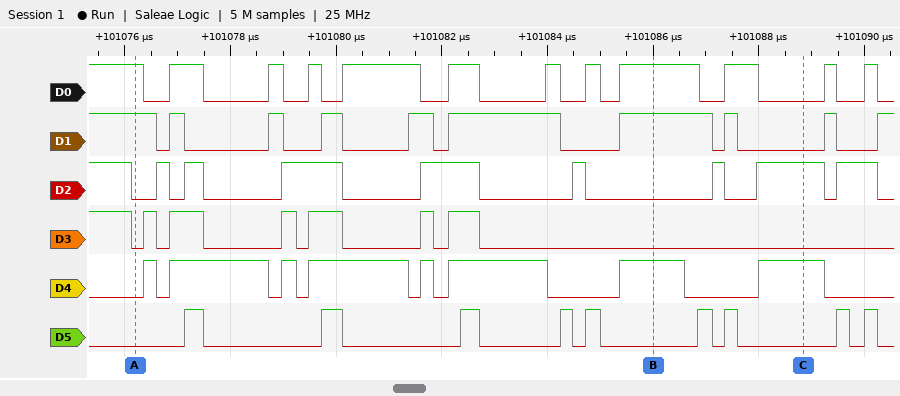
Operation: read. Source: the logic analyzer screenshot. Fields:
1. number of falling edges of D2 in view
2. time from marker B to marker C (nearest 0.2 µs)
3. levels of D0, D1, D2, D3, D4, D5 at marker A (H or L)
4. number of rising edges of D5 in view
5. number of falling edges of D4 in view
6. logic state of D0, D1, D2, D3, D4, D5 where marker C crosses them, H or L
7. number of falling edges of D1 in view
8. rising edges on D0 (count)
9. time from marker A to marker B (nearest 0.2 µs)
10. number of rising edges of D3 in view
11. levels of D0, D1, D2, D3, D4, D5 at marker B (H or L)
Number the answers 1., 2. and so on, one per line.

1. 9
2. 2.8 µs
3. D0=H, D1=H, D2=L, D3=L, D4=L, D5=L
4. 9
5. 8
6. D0=L, D1=L, D2=H, D3=L, D4=H, D5=L
7. 9
8. 11
9. 9.8 µs
10. 6
11. D0=H, D1=H, D2=L, D3=L, D4=H, D5=L
